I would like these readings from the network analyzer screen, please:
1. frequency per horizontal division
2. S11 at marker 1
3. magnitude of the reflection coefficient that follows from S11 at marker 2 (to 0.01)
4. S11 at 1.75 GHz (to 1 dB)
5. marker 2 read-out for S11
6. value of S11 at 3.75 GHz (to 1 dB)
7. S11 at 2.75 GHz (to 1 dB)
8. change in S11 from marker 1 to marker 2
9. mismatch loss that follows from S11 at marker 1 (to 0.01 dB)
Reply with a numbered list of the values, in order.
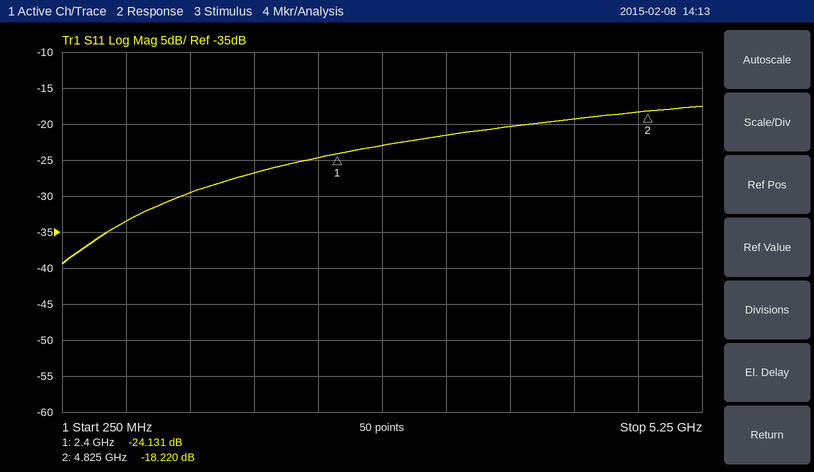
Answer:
1. 500 MHz
2. -24.131 dB
3. 0.12
4. -27 dB
5. -18.220 dB
6. -20 dB
7. -23 dB
8. 5.911 dB
9. 0.02 dB
